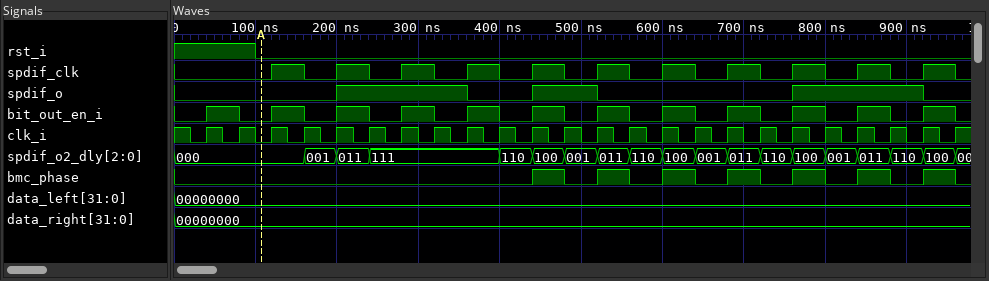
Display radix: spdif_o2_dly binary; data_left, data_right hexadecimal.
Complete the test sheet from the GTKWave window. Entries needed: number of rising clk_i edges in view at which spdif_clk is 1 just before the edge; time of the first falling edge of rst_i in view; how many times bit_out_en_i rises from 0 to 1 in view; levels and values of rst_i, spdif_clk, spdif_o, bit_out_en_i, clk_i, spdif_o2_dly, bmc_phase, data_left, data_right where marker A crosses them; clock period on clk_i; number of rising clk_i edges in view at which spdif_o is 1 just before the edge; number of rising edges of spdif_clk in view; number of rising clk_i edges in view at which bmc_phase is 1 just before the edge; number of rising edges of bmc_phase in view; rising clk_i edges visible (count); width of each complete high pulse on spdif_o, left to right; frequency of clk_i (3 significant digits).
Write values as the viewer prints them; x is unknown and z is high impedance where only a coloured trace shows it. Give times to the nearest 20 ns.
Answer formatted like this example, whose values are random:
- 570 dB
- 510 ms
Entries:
- 11
- 100 ns
- 12
- rst_i=0, spdif_clk=0, spdif_o=0, bit_out_en_i=0, clk_i=0, spdif_o2_dly=000, bmc_phase=0, data_left=00000000, data_right=00000000
- 40 ns
- 10
- 11
- 7
- 7
- 24
- 160 ns, 80 ns, 160 ns
- 25.0 MHz
